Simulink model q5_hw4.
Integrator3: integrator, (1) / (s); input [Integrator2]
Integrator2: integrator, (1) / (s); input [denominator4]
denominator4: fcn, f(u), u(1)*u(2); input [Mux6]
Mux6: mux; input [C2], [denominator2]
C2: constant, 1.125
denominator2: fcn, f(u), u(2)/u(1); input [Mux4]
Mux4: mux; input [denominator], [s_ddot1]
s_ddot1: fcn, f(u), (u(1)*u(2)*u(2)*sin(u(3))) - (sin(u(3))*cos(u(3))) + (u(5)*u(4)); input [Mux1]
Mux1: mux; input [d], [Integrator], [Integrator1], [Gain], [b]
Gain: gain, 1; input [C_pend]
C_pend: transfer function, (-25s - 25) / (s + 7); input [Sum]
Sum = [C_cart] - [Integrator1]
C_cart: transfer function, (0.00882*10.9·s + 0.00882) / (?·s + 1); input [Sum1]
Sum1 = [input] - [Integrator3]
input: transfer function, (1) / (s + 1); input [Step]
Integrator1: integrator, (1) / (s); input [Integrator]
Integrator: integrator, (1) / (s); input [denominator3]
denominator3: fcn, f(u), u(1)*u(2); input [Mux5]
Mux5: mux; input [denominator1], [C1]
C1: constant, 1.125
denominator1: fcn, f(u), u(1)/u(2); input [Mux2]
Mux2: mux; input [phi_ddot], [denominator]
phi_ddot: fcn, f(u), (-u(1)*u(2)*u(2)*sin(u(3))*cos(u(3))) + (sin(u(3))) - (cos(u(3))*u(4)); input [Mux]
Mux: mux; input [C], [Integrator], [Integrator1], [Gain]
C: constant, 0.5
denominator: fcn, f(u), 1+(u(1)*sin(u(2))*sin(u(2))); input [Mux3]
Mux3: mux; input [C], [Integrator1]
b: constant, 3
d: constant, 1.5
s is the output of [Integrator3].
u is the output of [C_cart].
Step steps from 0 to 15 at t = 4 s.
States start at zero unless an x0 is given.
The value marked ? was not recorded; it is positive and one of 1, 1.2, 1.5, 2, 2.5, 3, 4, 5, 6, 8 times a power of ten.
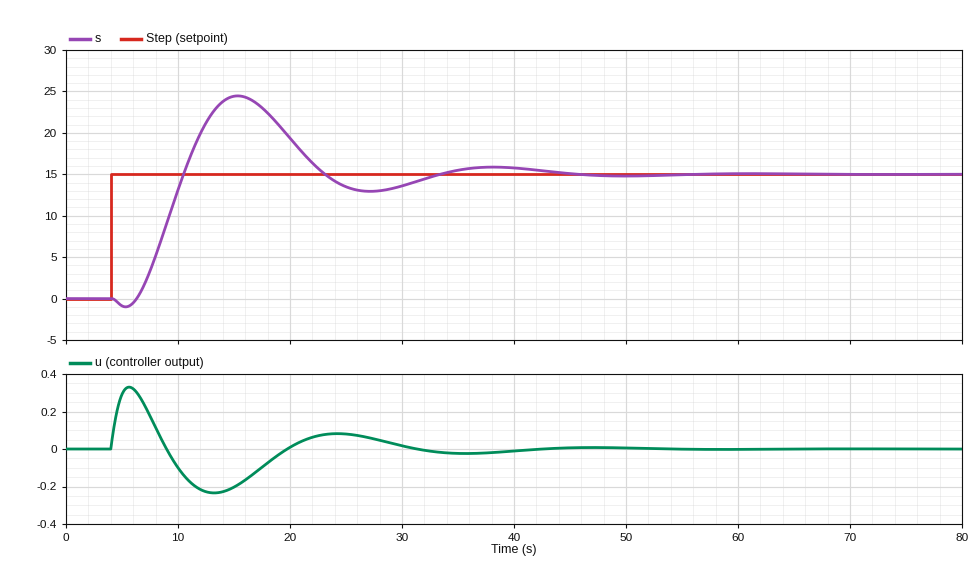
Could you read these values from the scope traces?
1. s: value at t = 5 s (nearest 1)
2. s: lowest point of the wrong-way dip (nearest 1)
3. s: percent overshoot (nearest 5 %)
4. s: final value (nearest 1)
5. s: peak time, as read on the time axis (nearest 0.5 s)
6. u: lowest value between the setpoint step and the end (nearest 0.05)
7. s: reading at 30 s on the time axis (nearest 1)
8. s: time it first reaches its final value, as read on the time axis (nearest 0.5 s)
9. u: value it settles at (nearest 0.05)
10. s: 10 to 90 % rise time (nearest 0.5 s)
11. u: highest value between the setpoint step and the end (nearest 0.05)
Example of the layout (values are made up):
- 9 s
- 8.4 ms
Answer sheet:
- -1
- -1
- 65 %
- 15
- 15.5 s
- -0.25
- 14
- 10.5 s
- 0.00
- 3.0 s
- 0.35
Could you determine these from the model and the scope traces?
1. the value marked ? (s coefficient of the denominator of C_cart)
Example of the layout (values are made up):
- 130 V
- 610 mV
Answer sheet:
- 3
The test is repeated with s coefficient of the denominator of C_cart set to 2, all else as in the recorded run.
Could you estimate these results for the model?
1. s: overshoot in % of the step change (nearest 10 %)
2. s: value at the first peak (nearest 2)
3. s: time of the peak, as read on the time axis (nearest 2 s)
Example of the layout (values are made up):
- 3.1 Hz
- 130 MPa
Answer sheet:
- 60 %
- 24
- 14 s
